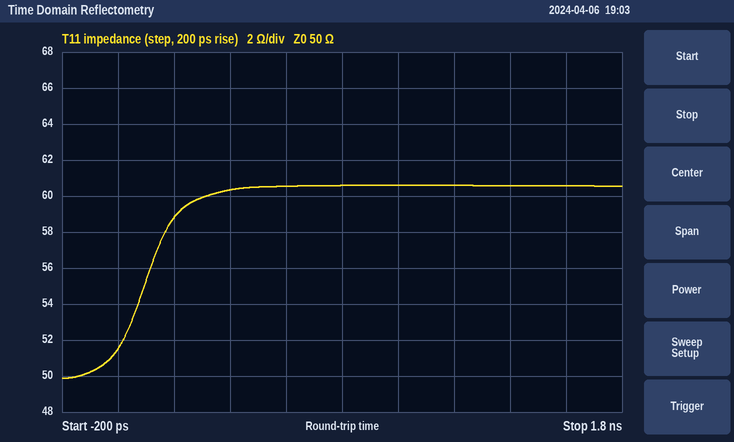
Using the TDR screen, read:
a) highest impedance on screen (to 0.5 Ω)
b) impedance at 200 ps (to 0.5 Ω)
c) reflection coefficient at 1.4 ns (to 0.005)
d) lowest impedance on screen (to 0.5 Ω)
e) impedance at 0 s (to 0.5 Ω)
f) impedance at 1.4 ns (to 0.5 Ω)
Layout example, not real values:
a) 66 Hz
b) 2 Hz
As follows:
a) 60.5 Ω
b) 59.0 Ω
c) +0.095
d) 50.0 Ω
e) 51.5 Ω
f) 60.5 Ω
